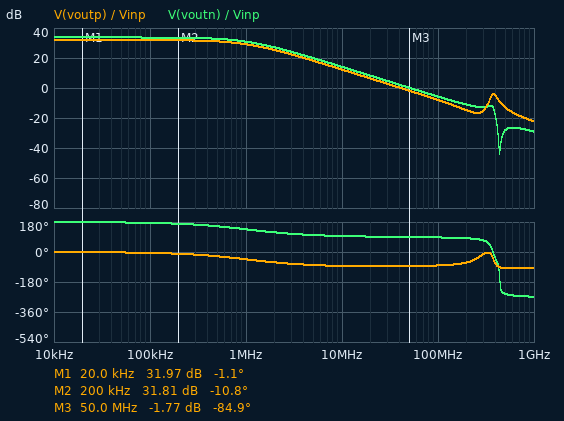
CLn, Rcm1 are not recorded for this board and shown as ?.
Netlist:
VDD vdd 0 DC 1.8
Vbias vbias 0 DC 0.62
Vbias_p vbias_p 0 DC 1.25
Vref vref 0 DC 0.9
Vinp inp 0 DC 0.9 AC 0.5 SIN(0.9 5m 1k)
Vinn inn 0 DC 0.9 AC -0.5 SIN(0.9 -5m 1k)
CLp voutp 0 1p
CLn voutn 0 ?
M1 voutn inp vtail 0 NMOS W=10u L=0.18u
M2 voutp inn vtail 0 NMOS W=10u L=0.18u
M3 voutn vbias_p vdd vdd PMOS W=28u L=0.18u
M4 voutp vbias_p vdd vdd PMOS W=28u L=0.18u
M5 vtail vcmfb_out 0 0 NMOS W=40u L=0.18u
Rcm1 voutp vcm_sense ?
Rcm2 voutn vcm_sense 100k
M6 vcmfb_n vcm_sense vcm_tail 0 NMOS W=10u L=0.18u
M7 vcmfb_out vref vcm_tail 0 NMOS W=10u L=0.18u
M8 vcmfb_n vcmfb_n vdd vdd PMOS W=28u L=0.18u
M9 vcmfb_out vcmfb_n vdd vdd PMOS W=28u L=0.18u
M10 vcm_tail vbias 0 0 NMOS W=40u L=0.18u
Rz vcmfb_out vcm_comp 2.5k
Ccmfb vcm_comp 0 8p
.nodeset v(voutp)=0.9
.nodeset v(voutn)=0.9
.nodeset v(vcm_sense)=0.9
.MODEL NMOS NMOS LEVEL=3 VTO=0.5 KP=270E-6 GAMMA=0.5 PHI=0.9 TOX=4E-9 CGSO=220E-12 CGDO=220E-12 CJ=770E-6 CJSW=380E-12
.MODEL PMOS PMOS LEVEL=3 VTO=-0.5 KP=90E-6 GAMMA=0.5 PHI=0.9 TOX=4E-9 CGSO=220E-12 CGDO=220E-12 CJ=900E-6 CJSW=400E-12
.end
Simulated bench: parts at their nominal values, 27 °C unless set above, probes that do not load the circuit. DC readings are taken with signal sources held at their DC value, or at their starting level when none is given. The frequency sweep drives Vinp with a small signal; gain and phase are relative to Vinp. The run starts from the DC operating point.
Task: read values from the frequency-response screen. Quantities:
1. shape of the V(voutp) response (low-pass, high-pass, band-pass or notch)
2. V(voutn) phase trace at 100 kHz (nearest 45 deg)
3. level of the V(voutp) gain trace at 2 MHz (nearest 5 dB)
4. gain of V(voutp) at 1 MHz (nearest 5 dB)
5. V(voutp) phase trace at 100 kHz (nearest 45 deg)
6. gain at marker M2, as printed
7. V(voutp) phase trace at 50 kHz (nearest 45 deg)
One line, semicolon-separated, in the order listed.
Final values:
low-pass; 180 deg; 25 dB; 30 dB; 0 deg; 31.81 dB; 0 deg
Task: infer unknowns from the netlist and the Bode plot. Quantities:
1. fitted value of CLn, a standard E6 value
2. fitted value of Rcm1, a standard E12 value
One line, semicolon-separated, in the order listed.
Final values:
2.2 pF; 82 kΩ
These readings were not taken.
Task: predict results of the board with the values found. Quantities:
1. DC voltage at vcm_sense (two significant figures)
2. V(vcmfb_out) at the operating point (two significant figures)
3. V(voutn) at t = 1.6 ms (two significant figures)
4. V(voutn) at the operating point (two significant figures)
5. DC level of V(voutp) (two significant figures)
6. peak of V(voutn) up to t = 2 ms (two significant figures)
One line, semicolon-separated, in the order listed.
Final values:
900 mV; 530 mV; 1.1 V; 900 mV; 900 mV; 1.2 V
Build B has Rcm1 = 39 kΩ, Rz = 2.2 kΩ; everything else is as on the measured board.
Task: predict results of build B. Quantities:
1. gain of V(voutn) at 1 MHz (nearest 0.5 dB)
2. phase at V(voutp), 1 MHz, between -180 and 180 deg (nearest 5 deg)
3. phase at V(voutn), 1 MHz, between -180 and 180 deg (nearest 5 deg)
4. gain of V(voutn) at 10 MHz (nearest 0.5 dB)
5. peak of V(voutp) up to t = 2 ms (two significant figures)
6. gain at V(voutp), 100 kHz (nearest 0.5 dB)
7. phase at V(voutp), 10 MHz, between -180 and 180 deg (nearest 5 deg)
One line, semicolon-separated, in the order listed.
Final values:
31.5 dB; -40 deg; 140 deg; 15.5 dB; 1.0 V; 25.5 dB; -80 deg
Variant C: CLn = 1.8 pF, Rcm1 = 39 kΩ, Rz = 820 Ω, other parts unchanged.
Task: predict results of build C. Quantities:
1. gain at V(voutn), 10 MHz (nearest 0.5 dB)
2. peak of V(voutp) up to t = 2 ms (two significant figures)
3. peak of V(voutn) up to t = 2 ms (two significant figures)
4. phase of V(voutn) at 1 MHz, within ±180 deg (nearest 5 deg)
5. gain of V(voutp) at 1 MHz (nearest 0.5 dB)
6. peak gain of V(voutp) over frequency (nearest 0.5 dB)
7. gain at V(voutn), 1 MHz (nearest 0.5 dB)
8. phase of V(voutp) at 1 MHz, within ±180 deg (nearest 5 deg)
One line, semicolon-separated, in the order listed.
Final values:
17.0 dB; 1.0 V; 1.2 V; 145 deg; 24.0 dB; 25.5 dB; 32.0 dB; -35 deg
